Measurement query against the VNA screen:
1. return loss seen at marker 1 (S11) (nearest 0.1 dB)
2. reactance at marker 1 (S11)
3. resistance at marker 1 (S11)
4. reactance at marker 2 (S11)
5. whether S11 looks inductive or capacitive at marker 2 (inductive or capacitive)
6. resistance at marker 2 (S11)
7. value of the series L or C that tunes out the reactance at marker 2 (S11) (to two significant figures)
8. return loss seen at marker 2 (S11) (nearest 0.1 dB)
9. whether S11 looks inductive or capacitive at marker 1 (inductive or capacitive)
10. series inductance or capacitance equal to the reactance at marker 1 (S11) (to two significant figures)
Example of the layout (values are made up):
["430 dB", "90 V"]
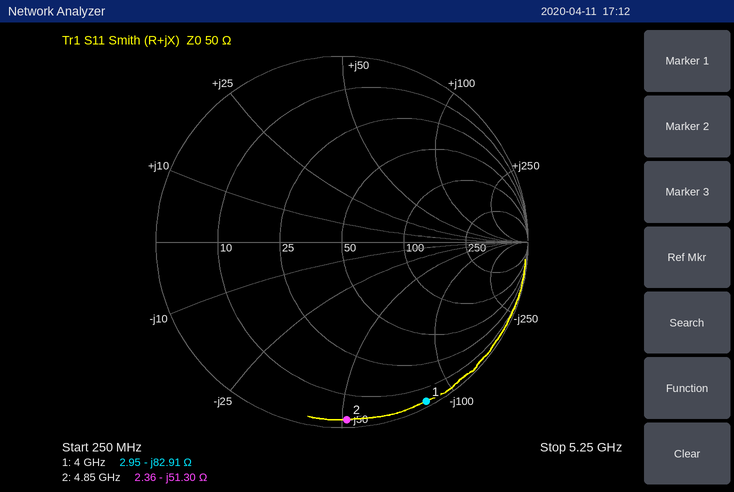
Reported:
["0.3 dB", "-82.91 Ω", "2.95 Ω", "-51.30 Ω", "capacitive", "2.36 Ω", "1.7 nH", "0.4 dB", "capacitive", "480 fF"]
